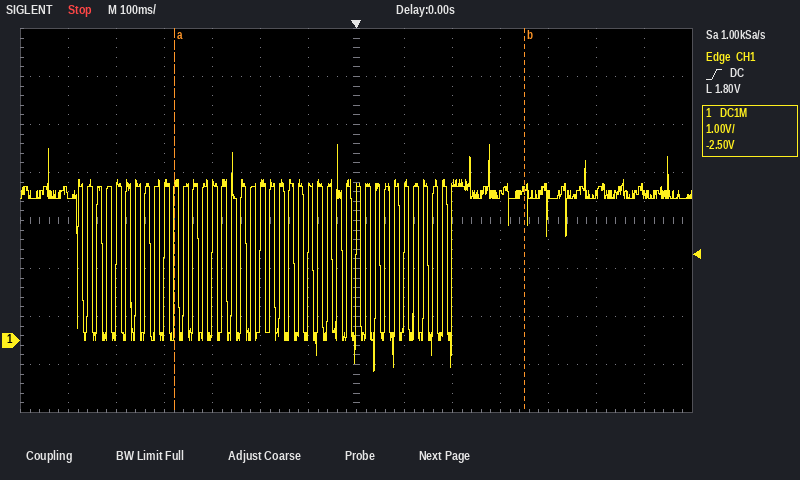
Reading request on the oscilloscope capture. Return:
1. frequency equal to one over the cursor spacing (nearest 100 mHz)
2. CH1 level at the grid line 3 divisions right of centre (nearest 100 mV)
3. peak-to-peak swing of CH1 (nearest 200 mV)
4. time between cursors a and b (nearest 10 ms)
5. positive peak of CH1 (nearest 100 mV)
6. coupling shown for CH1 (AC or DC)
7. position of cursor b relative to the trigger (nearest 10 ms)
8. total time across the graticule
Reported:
1.4 Hz
3.0 V
4.8 V
730 ms
4.1 V
DC
+350 ms
1.4 s
